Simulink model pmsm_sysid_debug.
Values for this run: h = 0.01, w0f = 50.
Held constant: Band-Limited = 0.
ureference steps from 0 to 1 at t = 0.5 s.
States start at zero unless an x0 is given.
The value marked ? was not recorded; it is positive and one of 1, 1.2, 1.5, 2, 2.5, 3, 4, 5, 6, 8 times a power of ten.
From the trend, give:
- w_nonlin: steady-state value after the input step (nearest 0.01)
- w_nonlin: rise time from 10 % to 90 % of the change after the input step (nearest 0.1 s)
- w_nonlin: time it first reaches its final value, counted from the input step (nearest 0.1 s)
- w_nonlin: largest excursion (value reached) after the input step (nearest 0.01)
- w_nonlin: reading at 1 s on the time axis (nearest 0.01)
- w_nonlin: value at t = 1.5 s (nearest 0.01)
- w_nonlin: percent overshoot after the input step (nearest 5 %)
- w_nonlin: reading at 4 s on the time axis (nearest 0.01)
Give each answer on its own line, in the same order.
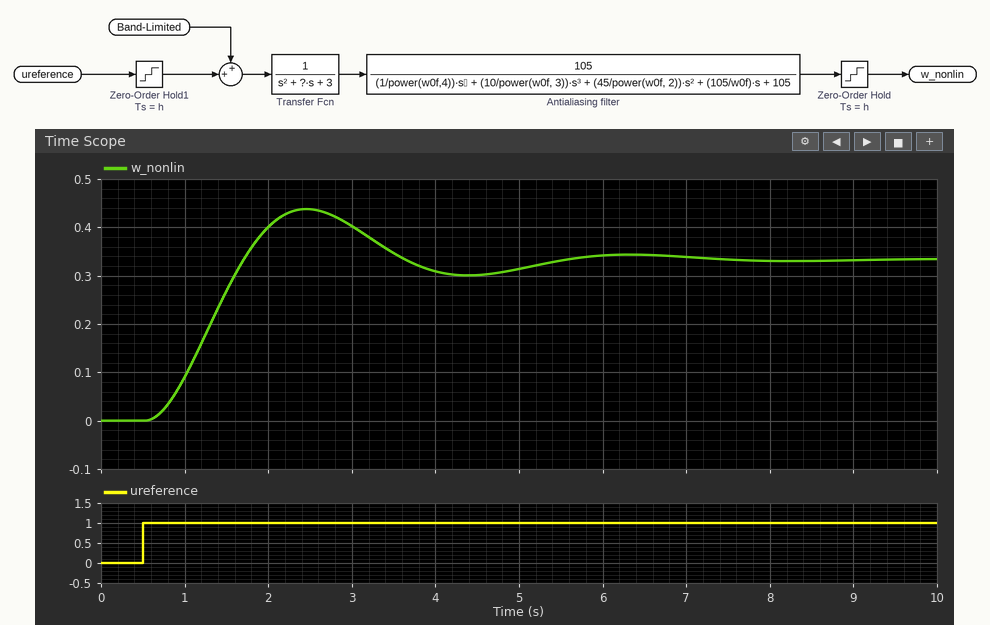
0.33
0.8 s
1.2 s
0.44
0.09
0.27
30 %
0.31
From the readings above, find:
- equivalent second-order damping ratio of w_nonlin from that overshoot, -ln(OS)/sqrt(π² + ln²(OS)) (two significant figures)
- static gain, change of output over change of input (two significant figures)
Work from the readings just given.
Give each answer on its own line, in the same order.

0.36
0.33
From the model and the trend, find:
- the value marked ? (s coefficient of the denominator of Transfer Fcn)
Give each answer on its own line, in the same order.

1.2
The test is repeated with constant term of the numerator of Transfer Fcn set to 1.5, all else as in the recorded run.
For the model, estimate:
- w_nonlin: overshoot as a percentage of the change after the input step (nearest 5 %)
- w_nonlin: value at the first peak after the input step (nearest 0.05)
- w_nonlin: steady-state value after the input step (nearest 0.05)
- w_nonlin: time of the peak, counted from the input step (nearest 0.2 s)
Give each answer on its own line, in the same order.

30 %
0.65
0.50
2.0 s
